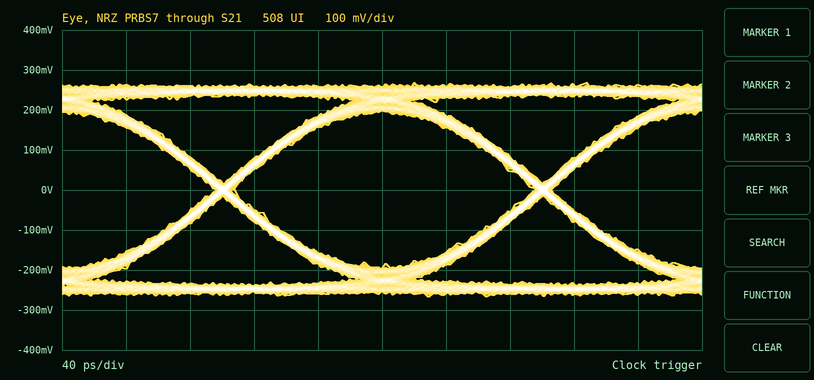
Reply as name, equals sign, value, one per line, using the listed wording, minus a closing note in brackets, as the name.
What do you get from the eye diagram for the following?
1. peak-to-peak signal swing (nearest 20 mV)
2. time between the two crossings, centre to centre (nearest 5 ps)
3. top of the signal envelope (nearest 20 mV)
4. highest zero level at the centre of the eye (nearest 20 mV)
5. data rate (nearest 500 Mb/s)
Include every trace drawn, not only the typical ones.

peak-to-peak signal swing = 540 mV
time between the two crossings, centre to centre = 200 ps
top of the signal envelope = 260 mV
highest zero level at the centre of the eye = -200 mV
data rate = 5.0 Gb/s
